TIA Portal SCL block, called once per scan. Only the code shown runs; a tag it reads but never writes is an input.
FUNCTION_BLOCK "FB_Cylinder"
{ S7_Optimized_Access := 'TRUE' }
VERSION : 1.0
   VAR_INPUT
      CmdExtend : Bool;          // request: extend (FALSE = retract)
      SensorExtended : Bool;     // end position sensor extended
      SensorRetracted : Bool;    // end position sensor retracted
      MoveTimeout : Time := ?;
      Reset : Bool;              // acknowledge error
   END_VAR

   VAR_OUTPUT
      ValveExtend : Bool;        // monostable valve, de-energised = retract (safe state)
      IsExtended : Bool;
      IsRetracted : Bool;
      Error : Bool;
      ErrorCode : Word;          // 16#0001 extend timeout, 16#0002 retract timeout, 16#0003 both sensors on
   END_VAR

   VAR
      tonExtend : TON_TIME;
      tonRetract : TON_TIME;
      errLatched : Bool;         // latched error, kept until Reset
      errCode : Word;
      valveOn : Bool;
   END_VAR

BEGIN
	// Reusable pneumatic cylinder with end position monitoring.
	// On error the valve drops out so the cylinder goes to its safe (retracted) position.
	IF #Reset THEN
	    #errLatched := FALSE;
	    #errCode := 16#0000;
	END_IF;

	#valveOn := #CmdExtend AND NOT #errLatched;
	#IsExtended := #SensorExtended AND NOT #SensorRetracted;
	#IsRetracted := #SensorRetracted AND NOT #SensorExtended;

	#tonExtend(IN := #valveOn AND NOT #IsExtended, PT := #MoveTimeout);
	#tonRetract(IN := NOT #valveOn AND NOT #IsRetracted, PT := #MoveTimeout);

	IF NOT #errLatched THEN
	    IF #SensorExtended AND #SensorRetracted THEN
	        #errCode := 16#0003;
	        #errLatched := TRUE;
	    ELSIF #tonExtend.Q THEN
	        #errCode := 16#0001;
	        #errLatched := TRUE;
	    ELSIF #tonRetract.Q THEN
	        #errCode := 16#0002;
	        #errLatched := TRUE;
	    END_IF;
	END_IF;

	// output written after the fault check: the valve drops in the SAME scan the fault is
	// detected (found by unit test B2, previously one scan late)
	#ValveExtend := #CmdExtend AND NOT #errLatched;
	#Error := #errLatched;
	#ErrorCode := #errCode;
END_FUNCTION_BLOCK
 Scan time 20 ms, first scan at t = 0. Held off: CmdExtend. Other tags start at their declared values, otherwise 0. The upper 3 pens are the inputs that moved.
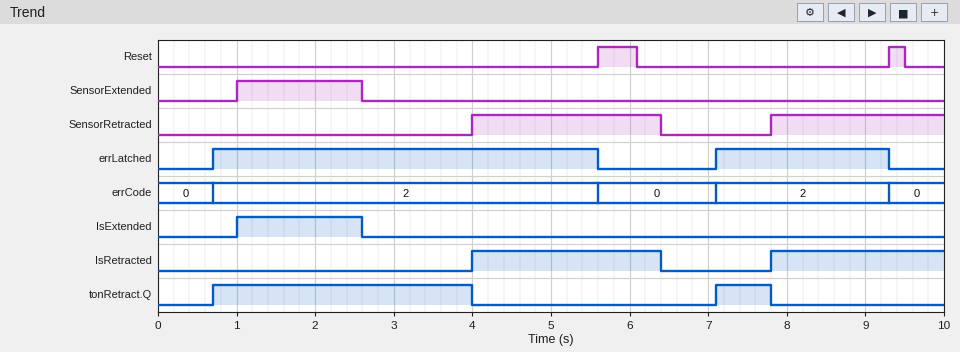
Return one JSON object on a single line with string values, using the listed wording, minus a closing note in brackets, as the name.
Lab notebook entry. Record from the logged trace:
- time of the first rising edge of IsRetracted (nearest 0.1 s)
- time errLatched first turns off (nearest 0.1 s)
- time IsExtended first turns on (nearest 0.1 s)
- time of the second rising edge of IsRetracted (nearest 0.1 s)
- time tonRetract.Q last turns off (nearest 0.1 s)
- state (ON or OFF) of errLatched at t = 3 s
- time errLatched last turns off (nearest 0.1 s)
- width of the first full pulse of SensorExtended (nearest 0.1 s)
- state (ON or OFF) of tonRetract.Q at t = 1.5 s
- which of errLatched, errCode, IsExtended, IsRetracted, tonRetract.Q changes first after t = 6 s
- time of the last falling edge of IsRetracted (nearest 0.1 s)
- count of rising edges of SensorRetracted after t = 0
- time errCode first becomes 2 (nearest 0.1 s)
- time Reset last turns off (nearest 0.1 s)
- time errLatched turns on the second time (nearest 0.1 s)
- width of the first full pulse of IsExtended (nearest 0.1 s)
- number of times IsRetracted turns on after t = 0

{"time of the first rising edge of IsRetracted": "4.0 s", "time errLatched first turns off": "5.6 s", "time IsExtended first turns on": "1.0 s", "time of the second rising edge of IsRetracted": "7.8 s", "time tonRetract.Q last turns off": "7.8 s", "state (ON or OFF) of errLatched at t = 3 s": "ON", "time errLatched last turns off": "9.3 s", "width of the first full pulse of SensorExtended": "1.6 s", "state (ON or OFF) of tonRetract.Q at t = 1.5 s": "ON", "which of errLatched, errCode, IsExtended, IsRetracted, tonRetract.Q changes first after t = 6 s": "IsRetracted", "time of the last falling edge of IsRetracted": "6.4 s", "count of rising edges of SensorRetracted after t = 0": "2", "time errCode first becomes 2": "0.7 s", "time Reset last turns off": "9.5 s", "time errLatched turns on the second time": "7.1 s", "width of the first full pulse of IsExtended": "1.6 s", "number of times IsRetracted turns on after t = 0": "2"}
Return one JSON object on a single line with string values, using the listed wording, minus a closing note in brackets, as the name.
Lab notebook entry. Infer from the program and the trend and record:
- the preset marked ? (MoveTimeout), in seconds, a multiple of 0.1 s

{"the preset marked ? (MoveTimeout), in seconds, a multiple of 0.1 s": "0.7 s"}
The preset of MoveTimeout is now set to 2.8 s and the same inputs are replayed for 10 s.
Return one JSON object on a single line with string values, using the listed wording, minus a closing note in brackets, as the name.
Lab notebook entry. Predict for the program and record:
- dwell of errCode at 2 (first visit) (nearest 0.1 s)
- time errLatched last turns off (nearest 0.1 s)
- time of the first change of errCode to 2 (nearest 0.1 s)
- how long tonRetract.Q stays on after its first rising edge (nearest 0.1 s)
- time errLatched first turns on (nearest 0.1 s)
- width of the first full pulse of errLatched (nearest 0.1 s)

{"dwell of errCode at 2 (first visit)": "2.8 s", "time errLatched last turns off": "5.6 s", "time of the first change of errCode to 2": "2.8 s", "how long tonRetract.Q stays on after its first rising edge": "1.2 s", "time errLatched first turns on": "2.8 s", "width of the first full pulse of errLatched": "2.8 s"}
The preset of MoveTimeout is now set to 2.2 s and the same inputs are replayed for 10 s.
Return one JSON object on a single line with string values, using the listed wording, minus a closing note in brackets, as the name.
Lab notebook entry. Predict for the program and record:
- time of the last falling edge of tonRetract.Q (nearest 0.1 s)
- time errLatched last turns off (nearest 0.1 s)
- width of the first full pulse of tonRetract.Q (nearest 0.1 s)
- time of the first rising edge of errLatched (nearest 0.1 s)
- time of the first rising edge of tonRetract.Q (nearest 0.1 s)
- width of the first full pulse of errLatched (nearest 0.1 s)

{"time of the last falling edge of tonRetract.Q": "4.0 s", "time errLatched last turns off": "5.6 s", "width of the first full pulse of tonRetract.Q": "1.8 s", "time of the first rising edge of errLatched": "2.2 s", "time of the first rising edge of tonRetract.Q": "2.2 s", "width of the first full pulse of errLatched": "3.4 s"}
